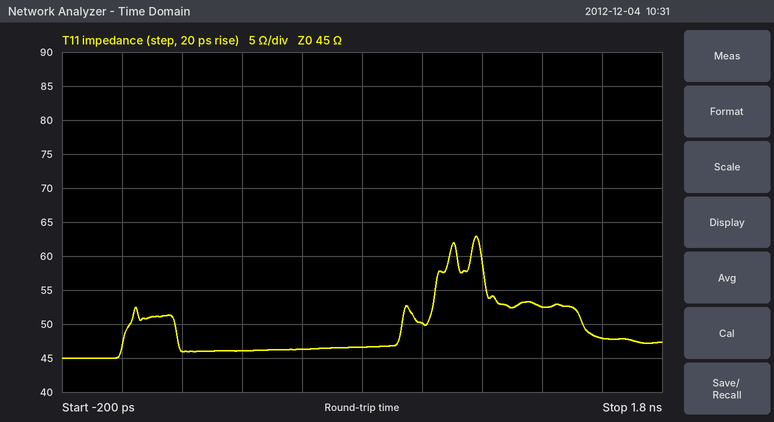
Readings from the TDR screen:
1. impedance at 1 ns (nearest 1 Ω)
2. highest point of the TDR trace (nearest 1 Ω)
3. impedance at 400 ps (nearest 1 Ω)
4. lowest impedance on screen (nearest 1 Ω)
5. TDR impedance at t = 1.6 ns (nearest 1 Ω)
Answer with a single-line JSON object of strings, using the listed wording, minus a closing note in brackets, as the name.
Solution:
{"impedance at 1 ns": "50 Ω", "highest point of the TDR trace": "63 Ω", "impedance at 400 ps": "46 Ω", "lowest impedance on screen": "45 Ω", "TDR impedance at t = 1.6 ns": "48 Ω"}
